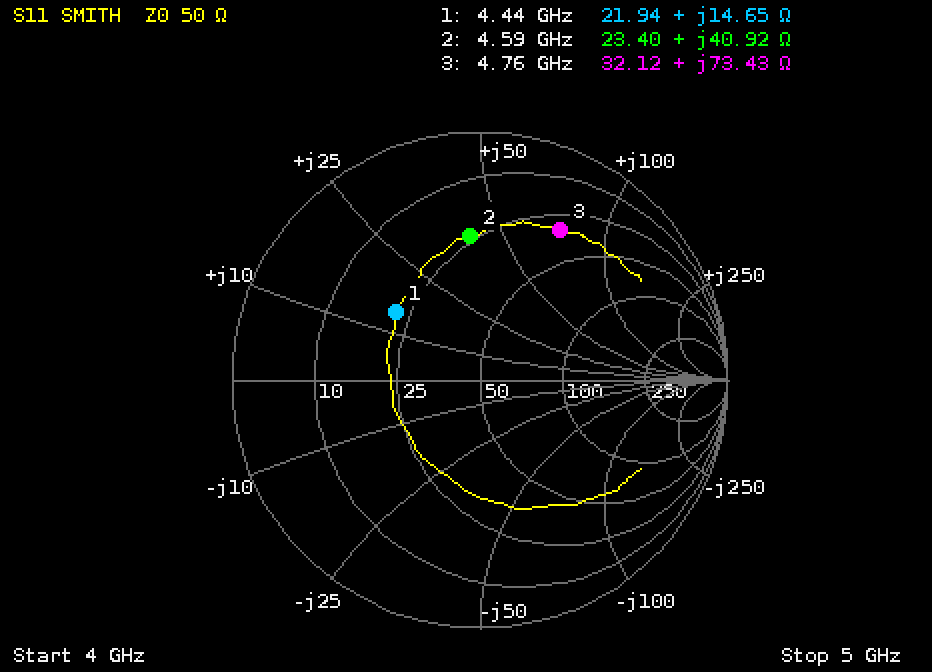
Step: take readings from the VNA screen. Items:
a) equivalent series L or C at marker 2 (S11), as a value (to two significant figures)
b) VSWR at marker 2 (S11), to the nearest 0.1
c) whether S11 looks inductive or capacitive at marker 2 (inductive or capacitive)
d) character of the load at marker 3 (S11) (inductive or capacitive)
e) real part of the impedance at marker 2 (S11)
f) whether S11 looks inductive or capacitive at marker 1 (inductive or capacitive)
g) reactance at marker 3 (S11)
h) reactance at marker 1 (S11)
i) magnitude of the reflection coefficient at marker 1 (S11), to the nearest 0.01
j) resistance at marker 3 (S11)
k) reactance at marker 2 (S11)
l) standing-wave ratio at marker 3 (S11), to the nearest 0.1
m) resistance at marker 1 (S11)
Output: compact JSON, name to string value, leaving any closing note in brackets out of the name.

{"equivalent series L or C at marker 2 (S11), as a value": "1.4 nH", "VSWR at marker 2 (S11), to the nearest 0.1": "3.8", "whether S11 looks inductive or capacitive at marker 2": "inductive", "character of the load at marker 3 (S11)": "inductive", "real part of the impedance at marker 2": "23.40 Ω", "whether S11 looks inductive or capacitive at marker 1": "inductive", "reactance at marker 3": "+73.43 Ω", "reactance at marker 1": "+14.65 Ω", "magnitude of the reflection coefficient at marker 1 (S11), to the nearest 0.01": "0.43", "resistance at marker 3": "32.12 Ω", "reactance at marker 2": "+40.92 Ω", "standing-wave ratio at marker 3 (S11), to the nearest 0.1": "5.4", "resistance at marker 1": "21.94 Ω"}
